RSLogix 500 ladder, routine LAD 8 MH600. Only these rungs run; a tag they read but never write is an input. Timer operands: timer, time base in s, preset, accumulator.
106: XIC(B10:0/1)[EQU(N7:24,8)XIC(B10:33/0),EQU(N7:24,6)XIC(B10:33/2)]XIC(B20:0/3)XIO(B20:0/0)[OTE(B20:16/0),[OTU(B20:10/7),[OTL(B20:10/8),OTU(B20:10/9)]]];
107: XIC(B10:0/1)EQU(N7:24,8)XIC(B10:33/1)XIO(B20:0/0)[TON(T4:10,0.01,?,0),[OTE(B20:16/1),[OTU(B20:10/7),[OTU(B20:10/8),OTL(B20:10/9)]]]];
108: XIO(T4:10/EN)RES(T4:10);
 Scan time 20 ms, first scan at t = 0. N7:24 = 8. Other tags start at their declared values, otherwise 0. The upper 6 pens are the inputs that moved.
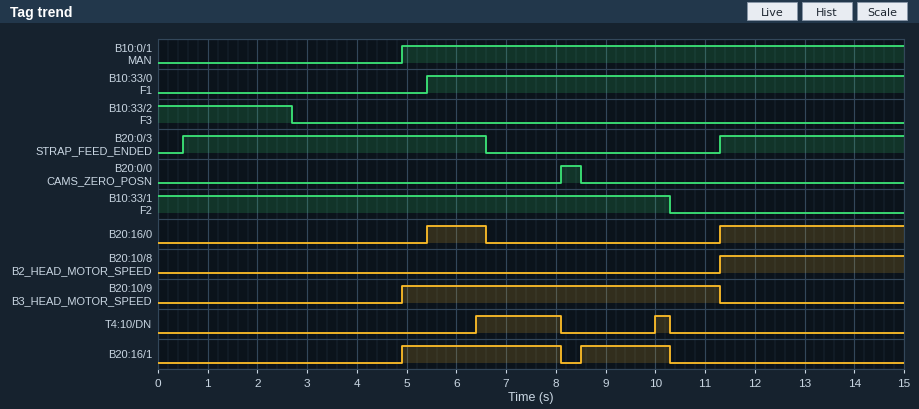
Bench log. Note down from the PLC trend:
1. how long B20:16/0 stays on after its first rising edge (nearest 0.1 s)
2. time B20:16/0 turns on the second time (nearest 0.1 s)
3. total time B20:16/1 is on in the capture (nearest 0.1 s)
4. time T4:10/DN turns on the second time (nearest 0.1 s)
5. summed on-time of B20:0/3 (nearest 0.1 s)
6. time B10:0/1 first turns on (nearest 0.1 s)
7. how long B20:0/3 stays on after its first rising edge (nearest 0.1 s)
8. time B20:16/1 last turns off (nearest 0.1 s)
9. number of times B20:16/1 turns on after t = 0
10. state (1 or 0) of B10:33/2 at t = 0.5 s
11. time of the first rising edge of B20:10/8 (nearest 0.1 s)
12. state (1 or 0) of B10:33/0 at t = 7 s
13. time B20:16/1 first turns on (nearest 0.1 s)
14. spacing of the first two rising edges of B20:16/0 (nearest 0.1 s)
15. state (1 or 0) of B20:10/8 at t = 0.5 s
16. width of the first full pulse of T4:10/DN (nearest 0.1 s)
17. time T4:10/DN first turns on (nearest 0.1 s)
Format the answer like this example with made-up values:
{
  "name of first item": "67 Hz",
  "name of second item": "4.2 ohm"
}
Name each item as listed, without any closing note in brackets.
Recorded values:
{
  "how long B20:16/0 stays on after its first rising edge": "1.2 s",
  "time B20:16/0 turns on the second time": "11.3 s",
  "total time B20:16/1 is on in the capture": "5.0 s",
  "time T4:10/DN turns on the second time": "10.0 s",
  "summed on-time of B20:0/3": "9.8 s",
  "time B10:0/1 first turns on": "4.9 s",
  "how long B20:0/3 stays on after its first rising edge": "6.1 s",
  "time B20:16/1 last turns off": "10.3 s",
  "number of times B20:16/1 turns on after t = 0": "2",
  "state (1 or 0) of B10:33/2 at t = 0.5 s": "1",
  "time of the first rising edge of B20:10/8": "11.3 s",
  "state (1 or 0) of B10:33/0 at t = 7 s": "1",
  "time B20:16/1 first turns on": "4.9 s",
  "spacing of the first two rising edges of B20:16/0": "5.9 s",
  "state (1 or 0) of B20:10/8 at t = 0.5 s": "0",
  "width of the first full pulse of T4:10/DN": "1.7 s",
  "time T4:10/DN first turns on": "6.4 s"
}
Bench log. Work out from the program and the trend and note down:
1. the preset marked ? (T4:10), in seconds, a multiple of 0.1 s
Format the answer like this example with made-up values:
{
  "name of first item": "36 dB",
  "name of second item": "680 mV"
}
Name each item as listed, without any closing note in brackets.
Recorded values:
{
  "the preset marked ? (T4:10), in seconds, a multiple of 0.1 s": "1.5 s"
}
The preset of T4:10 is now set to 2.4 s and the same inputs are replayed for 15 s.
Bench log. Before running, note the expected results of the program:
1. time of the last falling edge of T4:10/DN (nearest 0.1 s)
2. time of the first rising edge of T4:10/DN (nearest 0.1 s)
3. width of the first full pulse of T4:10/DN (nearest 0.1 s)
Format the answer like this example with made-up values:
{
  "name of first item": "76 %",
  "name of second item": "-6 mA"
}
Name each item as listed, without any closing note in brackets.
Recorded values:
{
  "time of the last falling edge of T4:10/DN": "8.1 s",
  "time of the first rising edge of T4:10/DN": "7.3 s",
  "width of the first full pulse of T4:10/DN": "0.8 s"
}
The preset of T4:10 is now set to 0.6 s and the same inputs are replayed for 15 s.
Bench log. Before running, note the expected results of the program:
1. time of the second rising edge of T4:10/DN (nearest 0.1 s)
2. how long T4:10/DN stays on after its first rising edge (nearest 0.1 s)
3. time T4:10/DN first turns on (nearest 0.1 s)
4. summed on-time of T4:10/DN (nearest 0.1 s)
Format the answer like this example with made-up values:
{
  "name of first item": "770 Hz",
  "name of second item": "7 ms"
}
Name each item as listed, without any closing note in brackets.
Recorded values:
{
  "time of the second rising edge of T4:10/DN": "9.1 s",
  "how long T4:10/DN stays on after its first rising edge": "2.6 s",
  "time T4:10/DN first turns on": "5.5 s",
  "summed on-time of T4:10/DN": "3.8 s"
}
